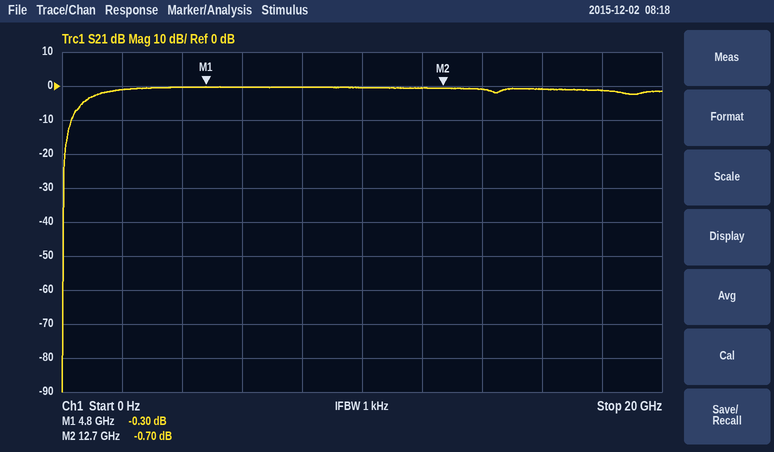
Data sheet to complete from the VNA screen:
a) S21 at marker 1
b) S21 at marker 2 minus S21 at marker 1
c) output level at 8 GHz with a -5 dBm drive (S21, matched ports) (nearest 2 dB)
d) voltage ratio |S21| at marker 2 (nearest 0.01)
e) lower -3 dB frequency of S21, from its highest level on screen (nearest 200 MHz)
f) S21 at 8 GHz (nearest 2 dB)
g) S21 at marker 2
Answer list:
-0.30 dB
-0.40 dB
-6 dBm
0.92
1.0 GHz
0 dB
-0.70 dB
